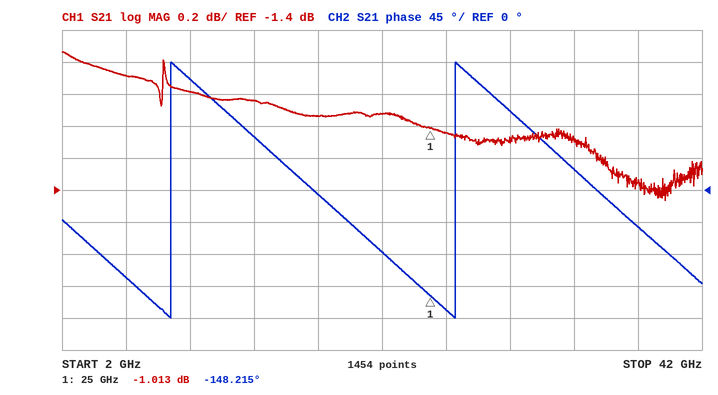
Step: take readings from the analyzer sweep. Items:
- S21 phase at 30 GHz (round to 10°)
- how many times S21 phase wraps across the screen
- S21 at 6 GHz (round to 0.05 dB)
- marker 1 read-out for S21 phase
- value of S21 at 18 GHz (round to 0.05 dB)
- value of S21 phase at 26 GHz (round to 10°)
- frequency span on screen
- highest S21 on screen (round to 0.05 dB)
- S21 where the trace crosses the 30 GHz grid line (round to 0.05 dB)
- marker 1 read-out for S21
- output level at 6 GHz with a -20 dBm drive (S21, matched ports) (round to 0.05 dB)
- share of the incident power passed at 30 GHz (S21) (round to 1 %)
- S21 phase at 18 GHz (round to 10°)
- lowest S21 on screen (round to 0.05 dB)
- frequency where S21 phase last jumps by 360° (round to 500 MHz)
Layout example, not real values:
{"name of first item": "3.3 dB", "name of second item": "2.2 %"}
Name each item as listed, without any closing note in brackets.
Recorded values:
{"S21 phase at 30 GHz": "110°", "how many times S21 phase wraps across the screen": "2", "S21 at 6 GHz": "-0.70 dB", "marker 1 read-out for S21 phase": "-148.215°", "value of S21 at 18 GHz": "-0.95 dB", "value of S21 phase at 26 GHz": "-170°", "frequency span on screen": "40 GHz", "highest S21 on screen": "-0.55 dB", "S21 where the trace crosses the 30 GHz grid line": "-1.10 dB", "marker 1 read-out for S21": "-1.013 dB", "output level at 6 GHz with a -20 dBm drive (S21, matched ports)": "-20.70 dBm", "share of the incident power passed at 30 GHz (S21)": "78 %", "S21 phase at 18 GHz": "-10°", "lowest S21 on screen": "-1.45 dB", "frequency where S21 phase last jumps by 360°": "26.5 GHz"}
